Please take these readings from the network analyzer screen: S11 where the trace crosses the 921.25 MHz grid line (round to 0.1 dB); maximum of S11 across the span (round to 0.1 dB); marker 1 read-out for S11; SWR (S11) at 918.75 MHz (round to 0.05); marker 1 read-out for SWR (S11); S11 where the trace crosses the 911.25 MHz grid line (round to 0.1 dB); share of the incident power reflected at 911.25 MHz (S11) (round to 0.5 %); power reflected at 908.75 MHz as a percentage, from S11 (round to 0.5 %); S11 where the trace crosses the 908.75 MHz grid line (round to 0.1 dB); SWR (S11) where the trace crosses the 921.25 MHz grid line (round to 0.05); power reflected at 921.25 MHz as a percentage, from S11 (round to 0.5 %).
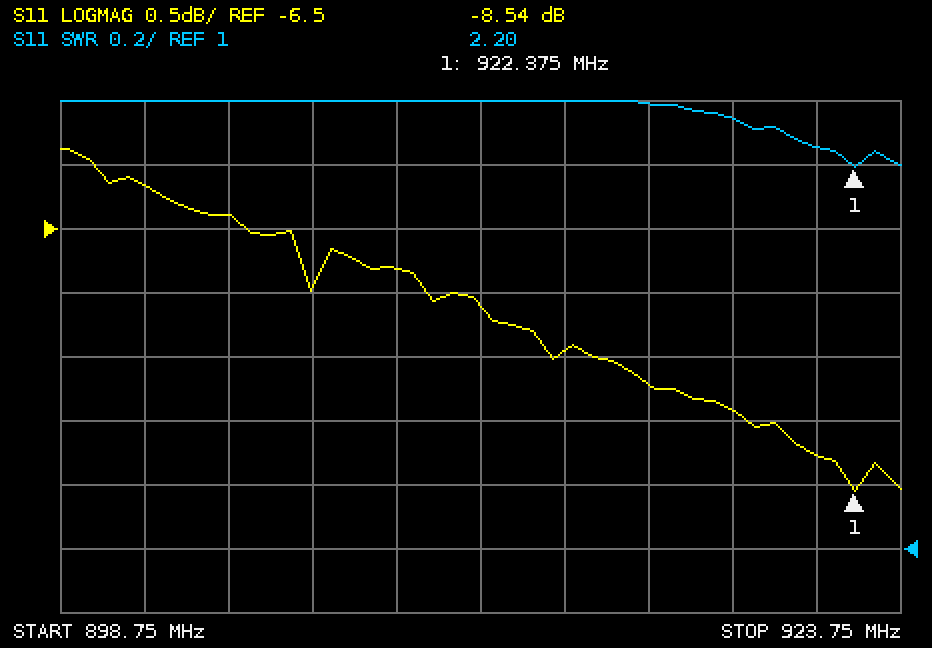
-8.3 dB
-5.9 dB
-8.54 dB
2.35
2.20
-7.1 dB
19.5 %
21.0 %
-6.8 dB
2.25
15.0 %
